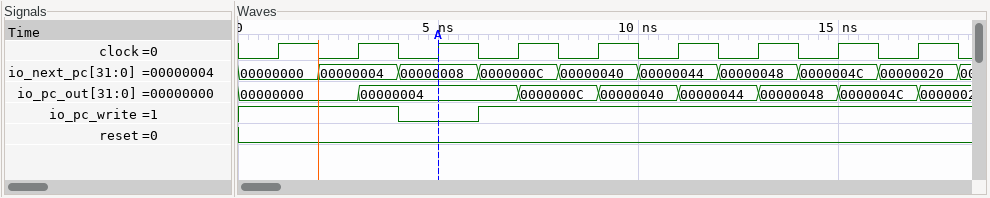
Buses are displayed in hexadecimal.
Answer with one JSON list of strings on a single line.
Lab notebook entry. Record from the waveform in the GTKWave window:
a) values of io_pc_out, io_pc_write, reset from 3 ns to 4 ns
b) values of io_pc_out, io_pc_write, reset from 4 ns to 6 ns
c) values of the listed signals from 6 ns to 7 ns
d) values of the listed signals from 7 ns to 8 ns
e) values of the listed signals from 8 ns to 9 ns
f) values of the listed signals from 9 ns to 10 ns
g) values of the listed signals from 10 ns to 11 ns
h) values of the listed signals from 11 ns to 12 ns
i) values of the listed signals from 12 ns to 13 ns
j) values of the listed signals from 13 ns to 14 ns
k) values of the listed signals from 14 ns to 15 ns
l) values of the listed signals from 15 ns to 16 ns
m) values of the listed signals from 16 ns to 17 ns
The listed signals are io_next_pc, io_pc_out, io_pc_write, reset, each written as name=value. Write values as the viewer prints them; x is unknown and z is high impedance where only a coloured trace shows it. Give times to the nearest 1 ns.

["io_pc_out=00000004, io_pc_write=1, reset=0", "io_pc_out=00000004, io_pc_write=0, reset=0", "io_next_pc=0000000C, io_pc_out=00000004, io_pc_write=1, reset=0", "io_next_pc=0000000C, io_pc_out=0000000C, io_pc_write=1, reset=0", "io_next_pc=00000040, io_pc_out=0000000C, io_pc_write=1, reset=0", "io_next_pc=00000040, io_pc_out=00000040, io_pc_write=1, reset=0", "io_next_pc=00000044, io_pc_out=00000040, io_pc_write=1, reset=0", "io_next_pc=00000044, io_pc_out=00000044, io_pc_write=1, reset=0", "io_next_pc=00000048, io_pc_out=00000044, io_pc_write=1, reset=0", "io_next_pc=00000048, io_pc_out=00000048, io_pc_write=1, reset=0", "io_next_pc=0000004C, io_pc_out=00000048, io_pc_write=1, reset=0", "io_next_pc=0000004C, io_pc_out=0000004C, io_pc_write=1, reset=0", "io_next_pc=00000020, io_pc_out=0000004C, io_pc_write=1, reset=0"]
